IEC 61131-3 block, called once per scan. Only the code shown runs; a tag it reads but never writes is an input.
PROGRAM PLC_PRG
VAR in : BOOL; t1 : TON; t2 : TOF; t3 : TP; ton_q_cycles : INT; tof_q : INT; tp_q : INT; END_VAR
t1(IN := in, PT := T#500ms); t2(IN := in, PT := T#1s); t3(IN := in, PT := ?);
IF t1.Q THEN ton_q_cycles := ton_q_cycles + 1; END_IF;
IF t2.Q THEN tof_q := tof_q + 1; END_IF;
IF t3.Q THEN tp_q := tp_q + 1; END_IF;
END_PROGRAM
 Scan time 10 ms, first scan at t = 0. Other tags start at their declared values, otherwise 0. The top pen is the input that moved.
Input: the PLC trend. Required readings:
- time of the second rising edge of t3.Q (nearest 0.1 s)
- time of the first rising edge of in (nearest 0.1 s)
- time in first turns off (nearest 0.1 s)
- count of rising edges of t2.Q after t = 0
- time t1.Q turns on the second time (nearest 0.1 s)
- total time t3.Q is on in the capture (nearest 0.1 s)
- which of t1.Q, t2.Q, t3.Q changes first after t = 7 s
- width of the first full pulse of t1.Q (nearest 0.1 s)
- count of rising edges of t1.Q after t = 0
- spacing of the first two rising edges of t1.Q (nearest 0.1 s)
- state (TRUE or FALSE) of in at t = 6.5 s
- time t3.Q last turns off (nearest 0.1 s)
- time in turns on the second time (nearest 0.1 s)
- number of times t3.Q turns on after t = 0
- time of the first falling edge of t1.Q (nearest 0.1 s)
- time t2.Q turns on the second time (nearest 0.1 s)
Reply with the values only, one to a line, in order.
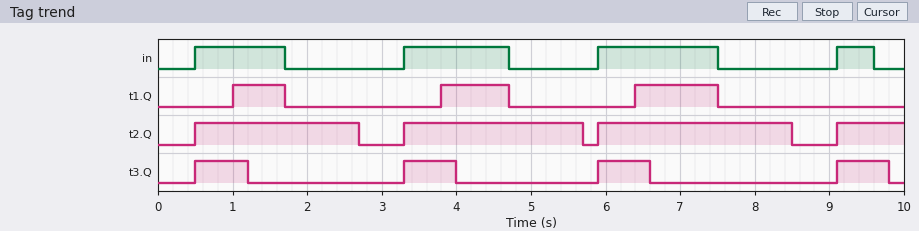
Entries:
3.3 s
0.5 s
1.7 s
4
3.8 s
2.8 s
t1.Q
0.7 s
3
2.8 s
TRUE
9.8 s
3.3 s
4
1.7 s
3.3 s
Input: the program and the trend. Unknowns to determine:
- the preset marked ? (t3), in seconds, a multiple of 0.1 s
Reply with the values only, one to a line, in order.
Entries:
0.7 s
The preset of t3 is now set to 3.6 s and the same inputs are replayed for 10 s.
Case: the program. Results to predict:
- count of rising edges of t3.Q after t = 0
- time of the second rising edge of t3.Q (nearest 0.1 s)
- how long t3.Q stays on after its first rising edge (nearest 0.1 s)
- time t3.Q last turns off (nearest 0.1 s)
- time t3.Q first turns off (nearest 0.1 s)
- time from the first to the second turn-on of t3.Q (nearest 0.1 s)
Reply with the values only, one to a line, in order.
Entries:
2
5.9 s
3.6 s
9.5 s
4.1 s
5.4 s
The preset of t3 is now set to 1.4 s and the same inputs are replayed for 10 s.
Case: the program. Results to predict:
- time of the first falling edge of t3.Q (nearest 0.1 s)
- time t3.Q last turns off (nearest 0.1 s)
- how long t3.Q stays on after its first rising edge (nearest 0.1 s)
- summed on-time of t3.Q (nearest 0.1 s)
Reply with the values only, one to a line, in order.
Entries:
1.9 s
7.3 s
1.4 s
5.1 s
